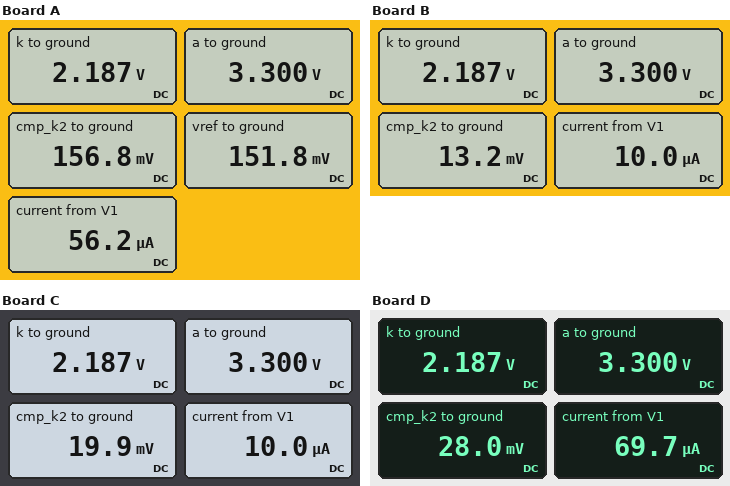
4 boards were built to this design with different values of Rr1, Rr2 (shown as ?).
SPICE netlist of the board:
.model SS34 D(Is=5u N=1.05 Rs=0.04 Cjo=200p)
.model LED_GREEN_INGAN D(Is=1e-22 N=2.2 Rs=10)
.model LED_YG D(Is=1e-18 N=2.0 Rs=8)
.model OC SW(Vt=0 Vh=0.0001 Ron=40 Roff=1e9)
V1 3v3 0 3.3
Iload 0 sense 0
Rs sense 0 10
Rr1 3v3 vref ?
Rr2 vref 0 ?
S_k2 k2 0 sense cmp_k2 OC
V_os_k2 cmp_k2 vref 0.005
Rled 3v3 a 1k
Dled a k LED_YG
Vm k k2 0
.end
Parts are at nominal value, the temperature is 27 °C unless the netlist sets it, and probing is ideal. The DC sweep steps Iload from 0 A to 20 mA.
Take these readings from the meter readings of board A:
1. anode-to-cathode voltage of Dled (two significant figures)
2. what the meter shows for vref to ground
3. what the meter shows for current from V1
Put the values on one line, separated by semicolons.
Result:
1.1 V; 151.8 mV; 56.2 µA
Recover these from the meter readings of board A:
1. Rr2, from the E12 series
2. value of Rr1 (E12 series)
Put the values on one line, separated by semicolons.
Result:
2.7 kΩ; 56 kΩ
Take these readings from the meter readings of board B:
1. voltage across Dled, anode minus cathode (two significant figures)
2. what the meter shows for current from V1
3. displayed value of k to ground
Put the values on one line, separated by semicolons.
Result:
1.1 V; 10.0 µA; 2.187 V
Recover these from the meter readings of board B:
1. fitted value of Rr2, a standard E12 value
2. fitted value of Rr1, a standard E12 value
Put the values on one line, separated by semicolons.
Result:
820 Ω; 330 kΩ
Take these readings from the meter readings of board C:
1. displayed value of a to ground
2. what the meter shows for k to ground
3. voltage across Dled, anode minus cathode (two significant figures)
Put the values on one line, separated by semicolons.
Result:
3.300 V; 2.187 V; 1.1 V
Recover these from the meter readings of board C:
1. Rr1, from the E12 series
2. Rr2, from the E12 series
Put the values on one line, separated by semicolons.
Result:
330 kΩ; 1.5 kΩ
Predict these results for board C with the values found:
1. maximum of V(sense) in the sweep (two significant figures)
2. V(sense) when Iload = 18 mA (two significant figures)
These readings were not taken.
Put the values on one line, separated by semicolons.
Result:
200 mV; 180 mV
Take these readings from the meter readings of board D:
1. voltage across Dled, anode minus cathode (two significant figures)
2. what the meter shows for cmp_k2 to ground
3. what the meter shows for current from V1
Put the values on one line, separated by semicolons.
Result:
1.1 V; 28.0 mV; 69.7 µA
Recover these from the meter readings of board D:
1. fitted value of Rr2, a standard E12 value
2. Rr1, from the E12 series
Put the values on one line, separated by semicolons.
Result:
330 Ω; 47 kΩ
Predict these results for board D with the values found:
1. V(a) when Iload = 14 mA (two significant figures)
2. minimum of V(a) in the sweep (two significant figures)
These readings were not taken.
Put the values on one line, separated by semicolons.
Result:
1.9 V; 1.9 V
